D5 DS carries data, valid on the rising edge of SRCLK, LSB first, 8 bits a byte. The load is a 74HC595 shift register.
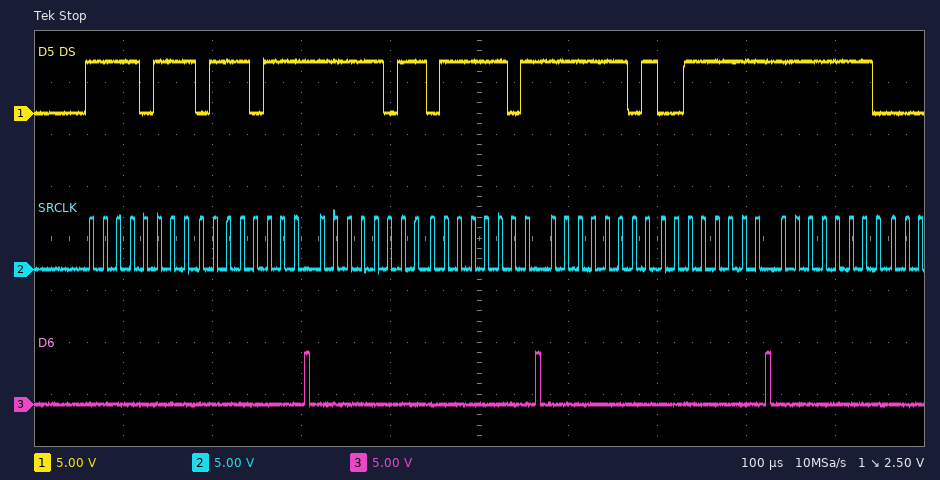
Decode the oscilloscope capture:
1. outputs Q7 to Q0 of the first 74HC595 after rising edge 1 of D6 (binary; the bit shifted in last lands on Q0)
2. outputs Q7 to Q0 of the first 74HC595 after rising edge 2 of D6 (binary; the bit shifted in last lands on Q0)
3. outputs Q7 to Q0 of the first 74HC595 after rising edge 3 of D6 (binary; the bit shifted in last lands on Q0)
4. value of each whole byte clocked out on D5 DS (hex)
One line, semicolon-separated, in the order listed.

01110111; 01111101; 00111111; EF EE DF BE BF FC 7F
